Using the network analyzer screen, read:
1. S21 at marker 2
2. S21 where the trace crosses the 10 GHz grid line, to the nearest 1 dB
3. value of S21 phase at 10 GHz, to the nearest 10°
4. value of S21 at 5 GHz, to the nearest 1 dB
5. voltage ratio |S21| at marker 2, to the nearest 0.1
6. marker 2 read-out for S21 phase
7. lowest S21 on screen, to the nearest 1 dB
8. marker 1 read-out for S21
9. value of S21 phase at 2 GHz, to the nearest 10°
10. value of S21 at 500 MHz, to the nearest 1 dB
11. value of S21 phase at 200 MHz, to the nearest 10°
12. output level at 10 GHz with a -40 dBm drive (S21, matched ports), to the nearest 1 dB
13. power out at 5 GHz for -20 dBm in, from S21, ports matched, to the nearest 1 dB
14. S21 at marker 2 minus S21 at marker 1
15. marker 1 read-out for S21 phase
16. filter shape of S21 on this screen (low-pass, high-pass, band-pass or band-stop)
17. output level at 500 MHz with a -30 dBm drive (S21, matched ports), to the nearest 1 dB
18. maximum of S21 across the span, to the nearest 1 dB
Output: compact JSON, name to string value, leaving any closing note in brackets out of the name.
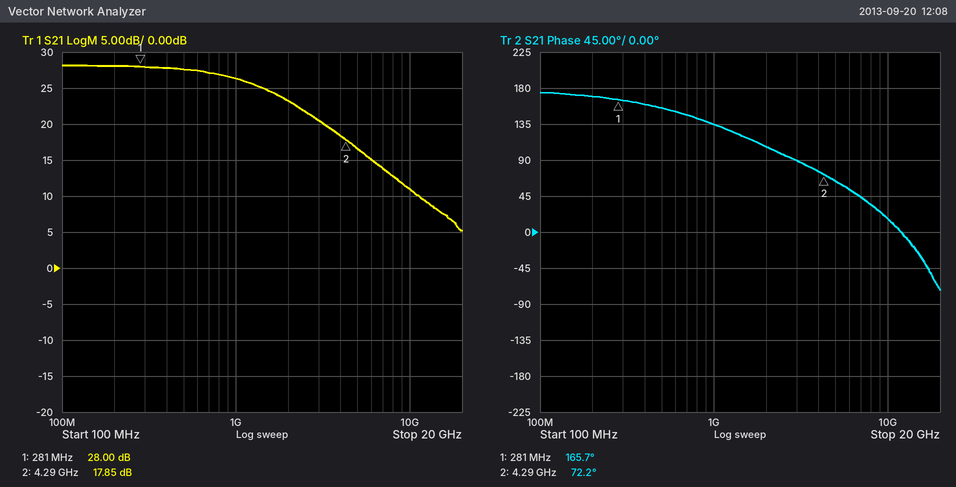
{"S21 at marker 2": "17.85 dB", "S21 where the trace crosses the 10 GHz grid line, to the nearest 1 dB": "11 dB", "value of S21 phase at 10 GHz, to the nearest 10°": "20°", "value of S21 at 5 GHz, to the nearest 1 dB": "17 dB", "voltage ratio |S21| at marker 2, to the nearest 0.1": "7.8", "marker 2 read-out for S21 phase": "72.2°", "lowest S21 on screen, to the nearest 1 dB": "5 dB", "marker 1 read-out for S21": "28.00 dB", "value of S21 phase at 2 GHz, to the nearest 10°": "110°", "value of S21 at 500 MHz, to the nearest 1 dB": "28 dB", "value of S21 phase at 200 MHz, to the nearest 10°": "170°", "output level at 10 GHz with a -40 dBm drive (S21, matched ports), to the nearest 1 dB": "-29 dBm", "power out at 5 GHz for -20 dBm in, from S21, ports matched, to the nearest 1 dB": "-3 dBm", "S21 at marker 2 minus S21 at marker 1": "-10.15 dB", "marker 1 read-out for S21 phase": "165.7°", "filter shape of S21 on this screen": "low-pass", "output level at 500 MHz with a -30 dBm drive (S21, matched ports), to the nearest 1 dB": "-2 dBm", "maximum of S21 across the span, to the nearest 1 dB": "28 dB"}
